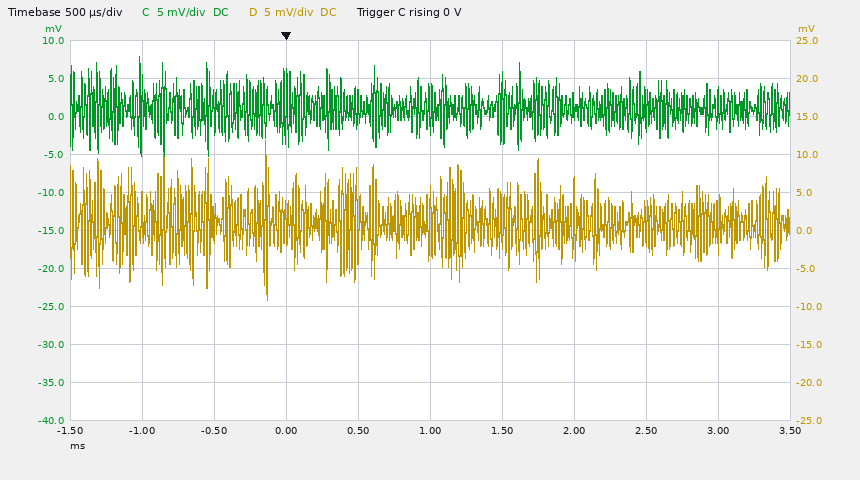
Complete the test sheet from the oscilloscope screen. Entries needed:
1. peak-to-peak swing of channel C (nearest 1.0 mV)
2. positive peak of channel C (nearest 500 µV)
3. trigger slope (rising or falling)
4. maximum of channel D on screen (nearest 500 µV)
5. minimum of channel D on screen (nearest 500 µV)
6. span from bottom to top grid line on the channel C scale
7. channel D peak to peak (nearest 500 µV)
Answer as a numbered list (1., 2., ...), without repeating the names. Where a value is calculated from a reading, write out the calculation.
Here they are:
1. 13.0 mV
2. 8.0 mV
3. rising
4. 12.0 mV
5. -9.0 mV
6. 50 mV
7. 12.0 mV − (-9.0 mV) = 21.0 mV
